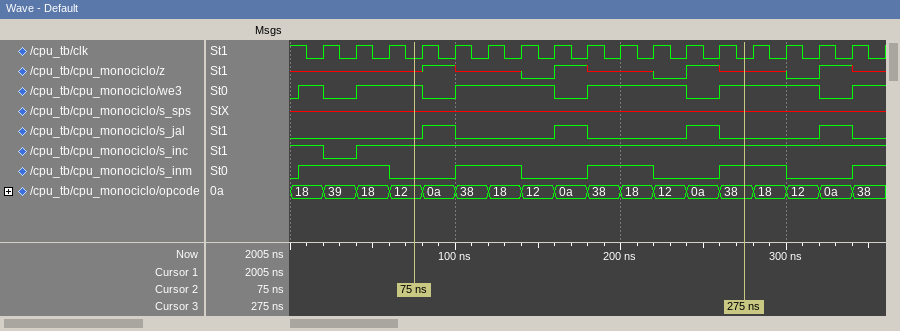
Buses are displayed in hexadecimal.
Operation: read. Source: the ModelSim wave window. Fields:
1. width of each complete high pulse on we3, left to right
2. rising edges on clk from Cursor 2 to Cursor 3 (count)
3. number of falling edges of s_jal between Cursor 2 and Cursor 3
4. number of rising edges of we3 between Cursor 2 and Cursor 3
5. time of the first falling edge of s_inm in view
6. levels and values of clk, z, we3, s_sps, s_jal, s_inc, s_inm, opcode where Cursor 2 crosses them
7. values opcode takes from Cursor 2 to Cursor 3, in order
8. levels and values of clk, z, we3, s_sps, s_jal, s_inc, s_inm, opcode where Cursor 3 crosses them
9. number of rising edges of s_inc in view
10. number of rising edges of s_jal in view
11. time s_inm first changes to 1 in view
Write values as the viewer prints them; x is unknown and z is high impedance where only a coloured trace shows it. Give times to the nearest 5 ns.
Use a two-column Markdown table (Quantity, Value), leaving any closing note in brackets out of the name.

| Quantity | Value |
|---|---|
| width of each complete high pulse on we3, left to right | 15 ns, 40 ns, 60 ns, 60 ns, 60 ns |
| rising edges on clk from Cursor 2 to Cursor 3 | 10 |
| number of falling edges of s_jal between Cursor 2 and Cursor 3 | 3 |
| number of rising edges of we3 between Cursor 2 and Cursor 3 | 3 |
| time of the first falling edge of s_inm in view | 60 ns |
| levels and values of clk, z, we3, s_sps, s_jal, s_inc, s_inm, opcode where Cursor 2 crosses them | clk=0, z=x, we3=1, s_sps=x, s_jal=0, s_inc=1, s_inm=0, opcode=12 |
| values opcode takes from Cursor 2 to Cursor 3, in order | 12, 0a, 38, 18, 12, 0a, 38, 18, 12, 0a, 38 |
| levels and values of clk, z, we3, s_sps, s_jal, s_inc, s_inm, opcode where Cursor 3 crosses them | clk=0, z=x, we3=1, s_sps=x, s_jal=0, s_inc=1, s_inm=1, opcode=38 |
| number of rising edges of s_inc in view | 1 |
| number of rising edges of s_jal in view | 4 |
| time s_inm first changes to 1 in view | 5 ns |
